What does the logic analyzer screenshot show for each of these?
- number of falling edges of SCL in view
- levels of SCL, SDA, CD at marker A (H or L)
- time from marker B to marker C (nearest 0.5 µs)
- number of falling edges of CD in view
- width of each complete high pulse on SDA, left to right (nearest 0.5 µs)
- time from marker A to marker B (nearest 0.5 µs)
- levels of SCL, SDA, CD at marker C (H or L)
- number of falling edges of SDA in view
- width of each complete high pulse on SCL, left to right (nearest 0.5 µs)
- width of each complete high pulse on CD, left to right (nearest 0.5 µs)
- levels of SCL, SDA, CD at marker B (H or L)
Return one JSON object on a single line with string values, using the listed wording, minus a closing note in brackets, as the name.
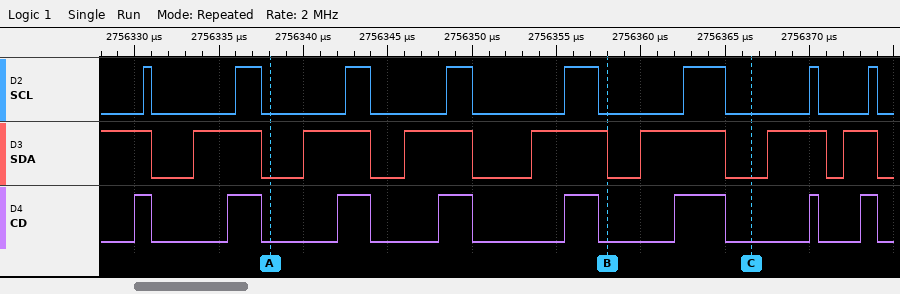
{"number of falling edges of SCL in view": "8", "levels of SCL, SDA, CD at marker A": "SCL=L, SDA=L, CD=L", "time from marker B to marker C": "8.5 µs", "number of falling edges of CD in view": "8", "width of each complete high pulse on SDA, left to right": "4 µs, 4 µs, 4 µs, 4.5 µs, 5 µs, 3.5 µs, 2 µs", "time from marker A to marker B": "20 µs", "levels of SCL, SDA, CD at marker C": "SCL=L, SDA=L, CD=L", "number of falling edges of SDA in view": "8", "width of each complete high pulse on SCL, left to right": "0.5 µs, 1.5 µs, 1.5 µs, 1.5 µs, 2 µs, 2.5 µs, 0.5 µs, 0.5 µs", "width of each complete high pulse on CD, left to right": "1 µs, 2 µs, 2 µs, 2 µs, 2 µs, 3 µs, 0.5 µs, 1 µs", "levels of SCL, SDA, CD at marker B": "SCL=L, SDA=L, CD=L"}
